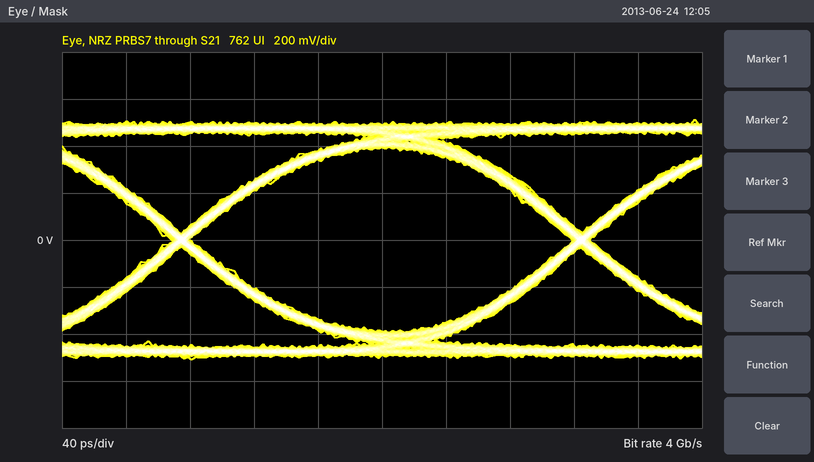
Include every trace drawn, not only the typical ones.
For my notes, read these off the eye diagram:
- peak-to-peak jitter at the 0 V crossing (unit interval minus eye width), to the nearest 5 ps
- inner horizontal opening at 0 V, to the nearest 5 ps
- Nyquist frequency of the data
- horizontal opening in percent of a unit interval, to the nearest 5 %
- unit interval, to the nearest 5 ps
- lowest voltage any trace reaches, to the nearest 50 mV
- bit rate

10 ps
240 ps
2 GHz
95 %
250 ps
-500 mV
4 Gb/s
